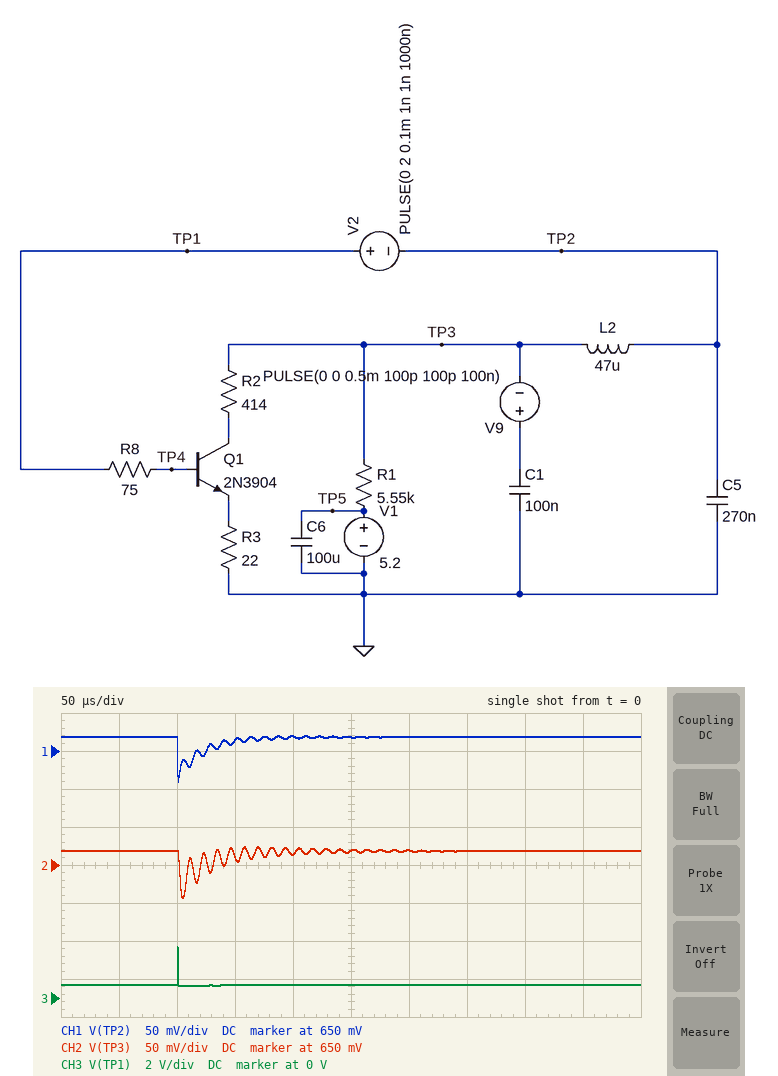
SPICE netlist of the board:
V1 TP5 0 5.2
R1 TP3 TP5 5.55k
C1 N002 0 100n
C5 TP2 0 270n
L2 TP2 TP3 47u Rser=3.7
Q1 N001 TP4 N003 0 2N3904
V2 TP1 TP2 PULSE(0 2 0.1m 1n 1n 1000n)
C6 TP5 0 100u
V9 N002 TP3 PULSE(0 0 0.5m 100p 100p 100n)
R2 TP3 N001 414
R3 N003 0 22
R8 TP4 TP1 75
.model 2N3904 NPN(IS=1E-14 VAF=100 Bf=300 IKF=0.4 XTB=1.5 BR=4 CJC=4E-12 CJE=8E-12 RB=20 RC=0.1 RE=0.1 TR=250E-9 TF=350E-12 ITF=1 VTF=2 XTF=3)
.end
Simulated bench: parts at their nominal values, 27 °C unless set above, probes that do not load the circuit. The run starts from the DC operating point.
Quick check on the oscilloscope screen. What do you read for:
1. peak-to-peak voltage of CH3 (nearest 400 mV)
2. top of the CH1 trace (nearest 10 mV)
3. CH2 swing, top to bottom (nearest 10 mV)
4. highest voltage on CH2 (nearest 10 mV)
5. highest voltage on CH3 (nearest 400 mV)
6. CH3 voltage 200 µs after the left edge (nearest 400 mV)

2.0 V
670 mV
70 mV
670 mV
2.8 V
800 mV
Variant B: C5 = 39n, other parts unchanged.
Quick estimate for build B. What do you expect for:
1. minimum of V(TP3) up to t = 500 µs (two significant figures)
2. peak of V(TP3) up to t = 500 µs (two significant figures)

500 mV
690 mV
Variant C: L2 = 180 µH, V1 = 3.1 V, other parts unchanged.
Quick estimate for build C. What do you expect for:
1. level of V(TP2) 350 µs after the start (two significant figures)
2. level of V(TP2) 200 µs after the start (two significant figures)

630 mV
650 mV
